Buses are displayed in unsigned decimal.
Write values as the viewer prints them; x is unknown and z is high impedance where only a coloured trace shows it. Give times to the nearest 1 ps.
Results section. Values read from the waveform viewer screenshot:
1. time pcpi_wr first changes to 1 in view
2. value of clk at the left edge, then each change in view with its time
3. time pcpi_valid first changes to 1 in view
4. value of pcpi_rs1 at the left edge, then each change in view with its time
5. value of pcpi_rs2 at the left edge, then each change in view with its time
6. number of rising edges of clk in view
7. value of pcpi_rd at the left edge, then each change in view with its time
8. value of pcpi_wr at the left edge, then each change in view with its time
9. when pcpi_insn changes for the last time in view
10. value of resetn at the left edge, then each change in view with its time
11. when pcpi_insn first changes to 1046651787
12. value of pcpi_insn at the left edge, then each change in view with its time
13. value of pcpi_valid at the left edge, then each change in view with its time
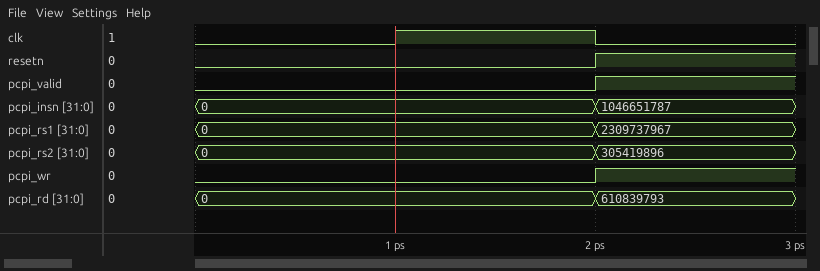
2 ps
0, 1 at 1 ps, 0 at 2 ps
2 ps
0, 2309737967 at 2 ps
0, 305419896 at 2 ps
1
0, 610839793 at 2 ps
0, 1 at 2 ps
2 ps
0, 1 at 2 ps
2 ps
0, 1046651787 at 2 ps
0, 1 at 2 ps
